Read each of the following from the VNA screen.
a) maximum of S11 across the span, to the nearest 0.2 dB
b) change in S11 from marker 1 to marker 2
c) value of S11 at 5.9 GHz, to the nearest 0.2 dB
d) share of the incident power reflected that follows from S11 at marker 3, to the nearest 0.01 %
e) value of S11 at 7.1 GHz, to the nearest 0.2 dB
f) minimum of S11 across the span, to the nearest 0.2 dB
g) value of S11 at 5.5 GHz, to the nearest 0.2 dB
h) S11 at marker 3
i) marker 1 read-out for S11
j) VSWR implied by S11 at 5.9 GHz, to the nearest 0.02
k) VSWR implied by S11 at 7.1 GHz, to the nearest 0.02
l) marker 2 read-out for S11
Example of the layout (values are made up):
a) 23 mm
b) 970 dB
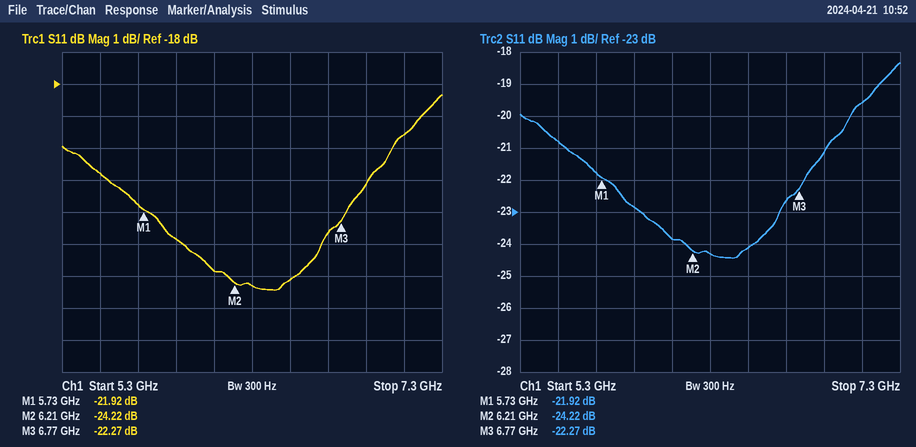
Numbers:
a) -18.4 dB
b) -2.30 dB
c) -22.8 dB
d) 0.59 %
e) -19.6 dB
f) -24.4 dB
g) -20.8 dB
h) -22.27 dB
i) -21.92 dB
j) 1.16
k) 1.24
l) -24.22 dB
